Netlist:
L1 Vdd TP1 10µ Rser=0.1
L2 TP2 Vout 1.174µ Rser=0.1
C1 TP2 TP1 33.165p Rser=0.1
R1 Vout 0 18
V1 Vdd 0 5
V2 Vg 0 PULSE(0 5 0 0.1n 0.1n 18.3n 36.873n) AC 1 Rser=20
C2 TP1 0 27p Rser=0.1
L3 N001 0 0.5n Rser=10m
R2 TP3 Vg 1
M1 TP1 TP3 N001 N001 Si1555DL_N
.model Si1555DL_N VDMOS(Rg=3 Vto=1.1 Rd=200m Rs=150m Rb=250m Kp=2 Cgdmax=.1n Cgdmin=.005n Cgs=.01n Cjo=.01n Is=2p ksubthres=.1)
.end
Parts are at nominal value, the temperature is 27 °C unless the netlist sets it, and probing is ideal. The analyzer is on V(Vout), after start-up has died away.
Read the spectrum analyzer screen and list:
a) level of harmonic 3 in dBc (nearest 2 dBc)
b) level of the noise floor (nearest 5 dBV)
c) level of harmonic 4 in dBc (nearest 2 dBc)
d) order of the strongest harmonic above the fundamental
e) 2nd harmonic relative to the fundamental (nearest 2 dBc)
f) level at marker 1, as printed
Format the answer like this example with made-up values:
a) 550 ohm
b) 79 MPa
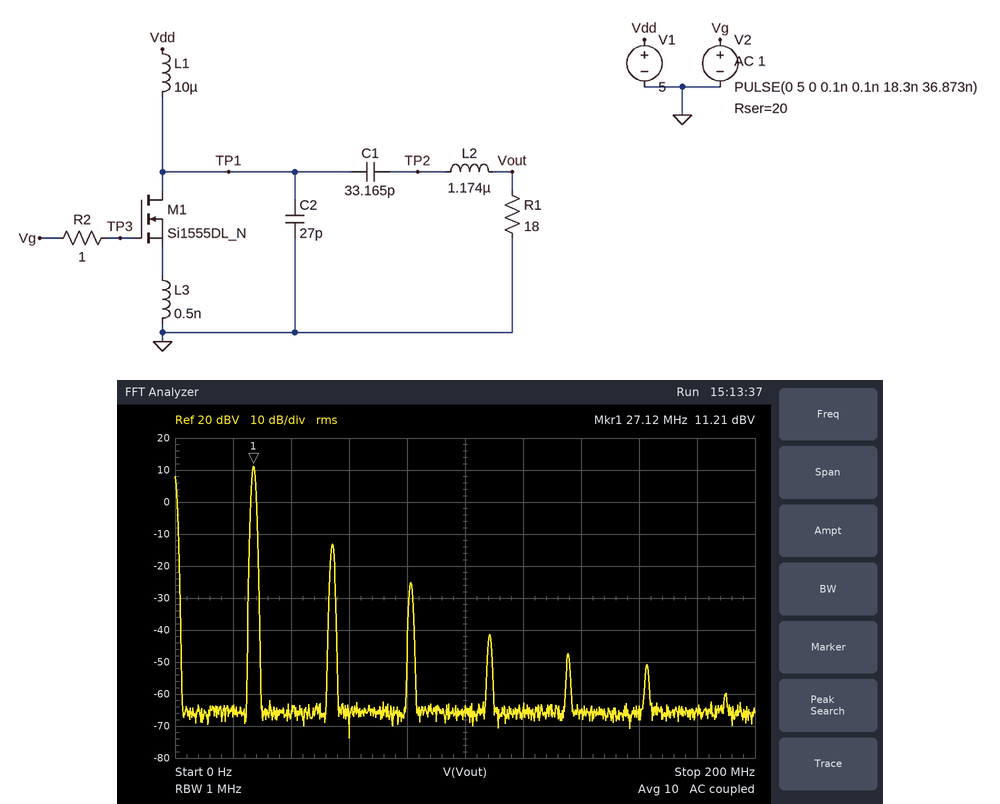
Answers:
a) -36 dBc
b) -65 dBV
c) -52 dBc
d) 2
e) -24 dBc
f) 11.21 dBV
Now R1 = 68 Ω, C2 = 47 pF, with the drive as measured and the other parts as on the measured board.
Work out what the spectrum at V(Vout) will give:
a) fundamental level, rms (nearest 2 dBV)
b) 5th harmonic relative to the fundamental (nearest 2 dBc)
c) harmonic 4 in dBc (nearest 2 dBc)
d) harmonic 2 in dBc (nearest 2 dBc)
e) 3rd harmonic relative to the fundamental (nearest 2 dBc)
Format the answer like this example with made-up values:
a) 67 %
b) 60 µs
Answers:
a) 14 dBV
b) -40 dBc
c) -36 dBc
d) -18 dBc
e) -32 dBc
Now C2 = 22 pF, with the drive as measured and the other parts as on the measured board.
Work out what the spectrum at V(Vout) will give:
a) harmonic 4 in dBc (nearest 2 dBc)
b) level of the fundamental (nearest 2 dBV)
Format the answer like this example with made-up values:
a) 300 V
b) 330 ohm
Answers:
a) -48 dBc
b) 12 dBV
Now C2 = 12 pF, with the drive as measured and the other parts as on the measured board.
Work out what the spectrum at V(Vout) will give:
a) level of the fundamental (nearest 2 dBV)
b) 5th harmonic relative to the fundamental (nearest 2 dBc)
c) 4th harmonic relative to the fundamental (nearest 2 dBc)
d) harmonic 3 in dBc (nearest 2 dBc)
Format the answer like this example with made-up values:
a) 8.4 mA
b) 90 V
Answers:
a) 12 dBV
b) -56 dBc
c) -42 dBc
d) -32 dBc
